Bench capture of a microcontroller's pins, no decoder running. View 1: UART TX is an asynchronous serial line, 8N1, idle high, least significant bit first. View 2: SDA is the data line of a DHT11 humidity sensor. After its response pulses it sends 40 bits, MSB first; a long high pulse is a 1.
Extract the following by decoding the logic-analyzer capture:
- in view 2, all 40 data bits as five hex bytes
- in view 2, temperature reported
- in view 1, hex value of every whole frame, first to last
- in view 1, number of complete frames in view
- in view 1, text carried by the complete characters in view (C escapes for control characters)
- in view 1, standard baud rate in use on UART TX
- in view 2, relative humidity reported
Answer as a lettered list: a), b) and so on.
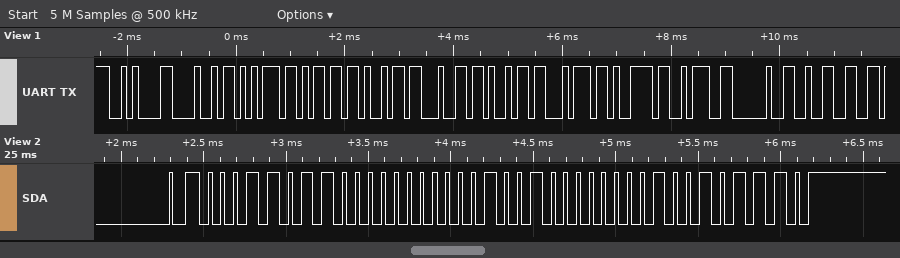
a) 1B 00 12 01 2E
b) 18.1 °C
c) 0A 48 75 6D 69 64 69 74 79 3A 20 32
d) 12
e) "\nHumidity: 2"
f) 9600 baud
g) 27 %
